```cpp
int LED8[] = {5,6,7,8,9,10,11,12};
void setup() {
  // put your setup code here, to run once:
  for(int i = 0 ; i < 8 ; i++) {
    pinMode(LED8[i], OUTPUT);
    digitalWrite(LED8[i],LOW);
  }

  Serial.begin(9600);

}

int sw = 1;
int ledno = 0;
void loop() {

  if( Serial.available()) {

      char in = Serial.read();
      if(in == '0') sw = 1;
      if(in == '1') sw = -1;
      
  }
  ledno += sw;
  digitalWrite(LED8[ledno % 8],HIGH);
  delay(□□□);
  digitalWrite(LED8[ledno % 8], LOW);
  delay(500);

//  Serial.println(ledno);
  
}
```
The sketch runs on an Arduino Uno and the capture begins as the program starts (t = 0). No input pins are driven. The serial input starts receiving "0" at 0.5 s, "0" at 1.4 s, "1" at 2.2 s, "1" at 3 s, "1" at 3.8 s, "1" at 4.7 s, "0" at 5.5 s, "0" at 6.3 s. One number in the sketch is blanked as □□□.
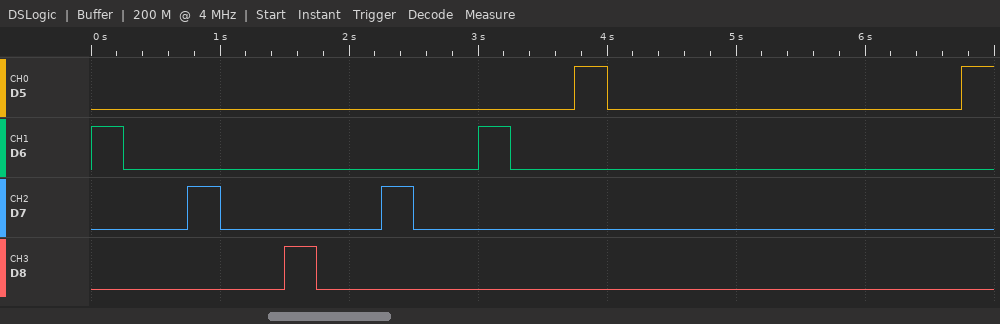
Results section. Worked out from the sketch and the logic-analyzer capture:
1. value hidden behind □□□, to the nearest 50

250
